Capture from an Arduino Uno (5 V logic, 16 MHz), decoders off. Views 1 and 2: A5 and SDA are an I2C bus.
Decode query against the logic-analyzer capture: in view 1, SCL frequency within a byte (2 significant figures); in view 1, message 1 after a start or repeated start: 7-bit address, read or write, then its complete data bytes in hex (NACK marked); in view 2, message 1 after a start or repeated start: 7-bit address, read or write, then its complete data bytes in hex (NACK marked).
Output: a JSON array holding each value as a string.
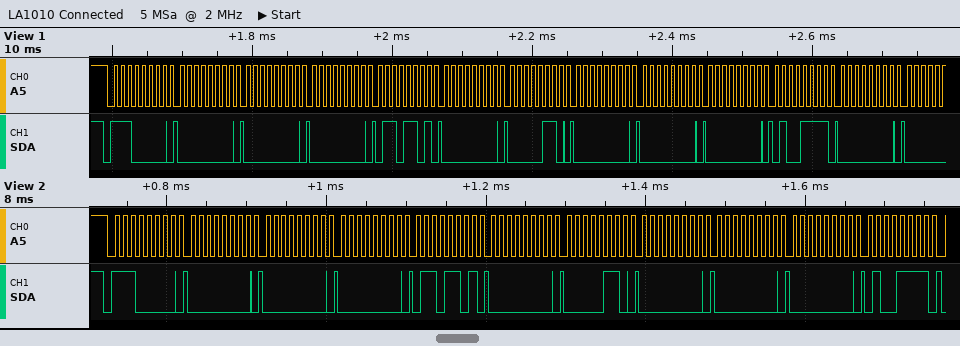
["100 kHz", "0x70 write: 00 00 00 6D 00 06 00 00 00 4F 00", "0x70 write: 00 00 00 6D 00 06 00 00 00 4F"]
